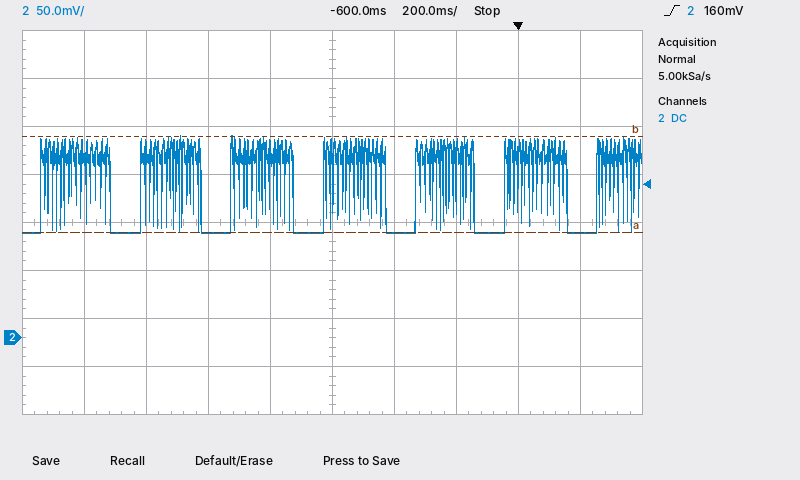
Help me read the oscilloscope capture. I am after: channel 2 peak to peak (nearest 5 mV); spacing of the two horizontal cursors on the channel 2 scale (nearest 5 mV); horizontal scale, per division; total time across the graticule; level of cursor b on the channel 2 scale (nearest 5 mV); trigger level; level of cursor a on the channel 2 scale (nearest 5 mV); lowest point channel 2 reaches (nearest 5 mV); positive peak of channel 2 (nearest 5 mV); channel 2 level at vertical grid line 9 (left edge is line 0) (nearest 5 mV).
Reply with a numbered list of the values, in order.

1. 100 mV
2. 100 mV
3. 200 ms
4. 2 s
5. 210 mV
6. 160 mV
7. 110 mV
8. 110 mV
9. 210 mV
10. 110 mV
